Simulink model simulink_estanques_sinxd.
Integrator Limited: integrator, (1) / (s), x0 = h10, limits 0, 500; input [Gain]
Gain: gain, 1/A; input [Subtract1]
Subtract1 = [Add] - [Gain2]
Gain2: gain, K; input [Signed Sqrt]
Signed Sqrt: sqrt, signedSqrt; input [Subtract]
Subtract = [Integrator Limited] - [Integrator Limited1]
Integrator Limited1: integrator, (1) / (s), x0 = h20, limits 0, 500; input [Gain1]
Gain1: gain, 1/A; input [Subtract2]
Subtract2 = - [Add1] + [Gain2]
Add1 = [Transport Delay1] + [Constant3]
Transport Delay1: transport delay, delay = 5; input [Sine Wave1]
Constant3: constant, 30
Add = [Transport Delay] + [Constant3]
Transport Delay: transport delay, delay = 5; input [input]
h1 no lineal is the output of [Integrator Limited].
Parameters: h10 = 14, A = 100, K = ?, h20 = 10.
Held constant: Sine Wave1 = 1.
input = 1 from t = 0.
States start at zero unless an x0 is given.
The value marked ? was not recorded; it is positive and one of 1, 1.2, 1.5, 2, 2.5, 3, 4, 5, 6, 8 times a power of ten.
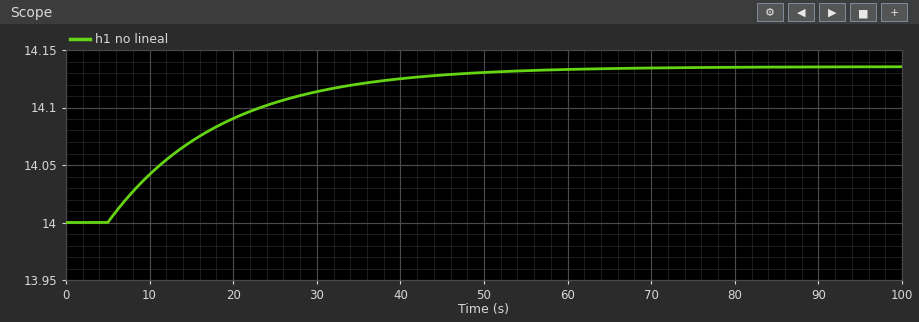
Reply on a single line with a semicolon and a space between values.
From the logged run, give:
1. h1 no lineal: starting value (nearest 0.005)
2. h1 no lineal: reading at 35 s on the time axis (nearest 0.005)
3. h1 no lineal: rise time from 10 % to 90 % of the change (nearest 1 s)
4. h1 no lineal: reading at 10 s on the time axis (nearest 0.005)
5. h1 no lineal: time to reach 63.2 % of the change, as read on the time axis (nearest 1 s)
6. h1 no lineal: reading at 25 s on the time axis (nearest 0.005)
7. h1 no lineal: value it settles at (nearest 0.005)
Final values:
14.000; 14.120; 30 s; 14.040; 19 s; 14.105; 14.135
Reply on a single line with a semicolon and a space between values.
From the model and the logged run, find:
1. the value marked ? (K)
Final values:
15
